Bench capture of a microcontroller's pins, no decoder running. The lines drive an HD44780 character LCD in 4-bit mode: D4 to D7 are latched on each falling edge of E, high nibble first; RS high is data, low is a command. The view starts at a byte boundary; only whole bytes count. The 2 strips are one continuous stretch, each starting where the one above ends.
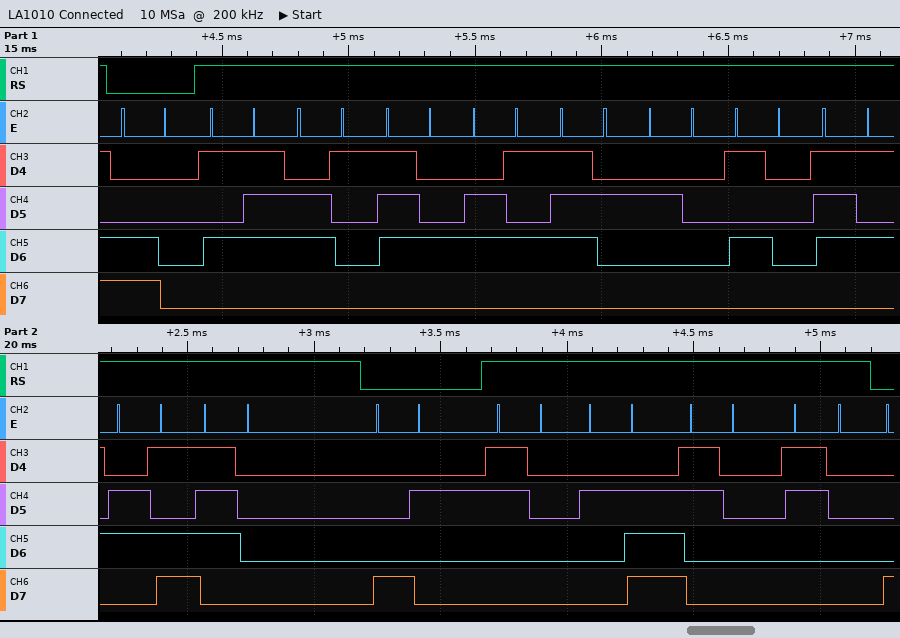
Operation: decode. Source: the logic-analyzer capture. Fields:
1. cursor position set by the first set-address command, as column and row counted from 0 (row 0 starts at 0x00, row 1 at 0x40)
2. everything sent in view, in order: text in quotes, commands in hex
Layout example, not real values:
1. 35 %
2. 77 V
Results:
1. column 0, row 1
2. 0xC0 "Water Pump" 0x82 "0.00"
